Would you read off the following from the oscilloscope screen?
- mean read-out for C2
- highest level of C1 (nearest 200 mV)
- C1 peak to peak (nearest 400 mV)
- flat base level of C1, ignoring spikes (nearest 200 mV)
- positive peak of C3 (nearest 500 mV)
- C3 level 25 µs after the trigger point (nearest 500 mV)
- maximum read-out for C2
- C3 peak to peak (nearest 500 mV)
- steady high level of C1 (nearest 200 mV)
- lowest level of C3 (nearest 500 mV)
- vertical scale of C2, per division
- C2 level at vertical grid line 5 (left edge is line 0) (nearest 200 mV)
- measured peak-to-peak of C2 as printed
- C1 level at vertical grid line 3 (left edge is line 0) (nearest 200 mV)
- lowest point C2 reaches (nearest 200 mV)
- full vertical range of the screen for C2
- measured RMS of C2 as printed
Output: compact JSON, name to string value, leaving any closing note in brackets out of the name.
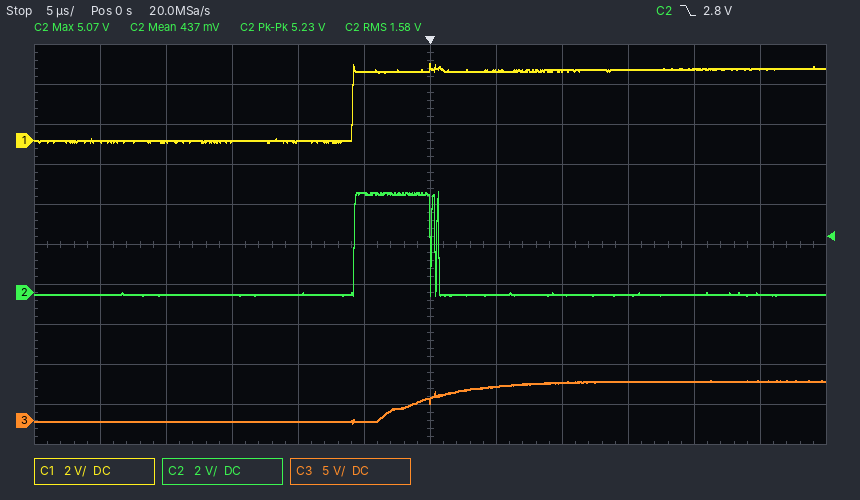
{"mean read-out for C2": "437 mV", "highest level of C1": "3.8 V", "C1 peak to peak": "4.0 V", "flat base level of C1, ignoring spikes": "0.0 V", "positive peak of C3": "5.0 V", "C3 level 25 µs after the trigger point": "5.0 V", "maximum read-out for C2": "5.07 V", "C3 peak to peak": "5.5 V", "steady high level of C1": "3.6 V", "lowest level of C3": "-500 mV", "vertical scale of C2, per division": "2 V", "C2 level at vertical grid line 5 (left edge is line 0)": "5.0 V", "measured peak-to-peak of C2 as printed": "5.23 V", "C1 level at vertical grid line 3 (left edge is line 0)": "0.0 V", "lowest point C2 reaches": "-200 mV", "full vertical range of the screen for C2": "20 V", "measured RMS of C2 as printed": "1.58 V"}
